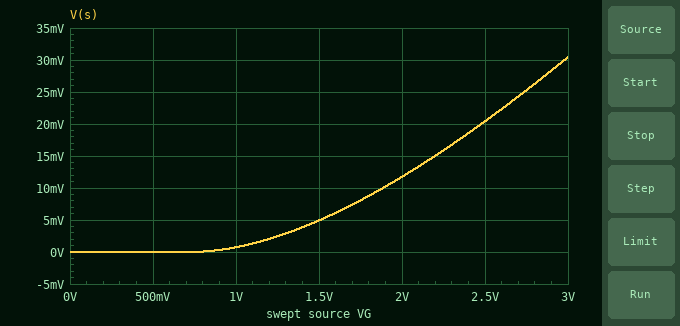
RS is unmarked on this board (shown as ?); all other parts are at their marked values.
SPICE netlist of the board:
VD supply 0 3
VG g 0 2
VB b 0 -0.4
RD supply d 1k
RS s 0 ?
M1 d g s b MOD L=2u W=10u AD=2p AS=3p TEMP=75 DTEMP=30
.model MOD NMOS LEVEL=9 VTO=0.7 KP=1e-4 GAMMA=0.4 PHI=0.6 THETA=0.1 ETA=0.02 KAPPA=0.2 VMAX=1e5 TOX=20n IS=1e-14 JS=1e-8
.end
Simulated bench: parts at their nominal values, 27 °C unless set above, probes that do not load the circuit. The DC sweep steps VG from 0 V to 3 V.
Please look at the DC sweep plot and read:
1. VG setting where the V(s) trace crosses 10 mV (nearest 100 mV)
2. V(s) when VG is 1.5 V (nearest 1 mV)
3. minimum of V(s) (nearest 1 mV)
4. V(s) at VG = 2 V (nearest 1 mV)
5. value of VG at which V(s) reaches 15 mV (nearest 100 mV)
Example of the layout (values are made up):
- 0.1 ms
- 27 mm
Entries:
- 1.9 V
- 5 mV
- 0 V
- 12 mV
- 2.2 V
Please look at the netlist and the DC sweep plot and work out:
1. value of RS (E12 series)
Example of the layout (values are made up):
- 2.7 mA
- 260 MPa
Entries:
- 56 Ω
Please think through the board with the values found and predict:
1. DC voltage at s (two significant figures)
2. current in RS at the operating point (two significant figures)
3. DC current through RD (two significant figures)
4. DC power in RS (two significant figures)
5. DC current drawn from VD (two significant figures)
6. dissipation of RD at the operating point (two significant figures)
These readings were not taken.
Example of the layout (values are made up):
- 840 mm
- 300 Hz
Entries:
- 12 mV
- 210 µA
- 210 µA
- 2.5 µW
- 210 µA
- 44 µW
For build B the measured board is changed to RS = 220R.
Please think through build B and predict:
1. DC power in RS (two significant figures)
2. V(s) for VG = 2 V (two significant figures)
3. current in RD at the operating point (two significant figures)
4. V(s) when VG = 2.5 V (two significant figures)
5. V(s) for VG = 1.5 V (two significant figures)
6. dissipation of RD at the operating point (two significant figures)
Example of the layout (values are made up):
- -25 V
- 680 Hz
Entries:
- 8.7 µW
- 44 mV
- 200 µA
- 75 mV
- 19 mV
- 40 µW
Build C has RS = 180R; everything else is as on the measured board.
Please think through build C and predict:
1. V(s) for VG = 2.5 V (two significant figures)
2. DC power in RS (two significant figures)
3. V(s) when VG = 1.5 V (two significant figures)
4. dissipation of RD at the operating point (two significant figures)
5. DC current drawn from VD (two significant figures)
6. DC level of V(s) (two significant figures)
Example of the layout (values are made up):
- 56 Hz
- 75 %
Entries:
- 63 mV
- 7.3 µW
- 15 mV
- 41 µW
- 200 µA
- 36 mV
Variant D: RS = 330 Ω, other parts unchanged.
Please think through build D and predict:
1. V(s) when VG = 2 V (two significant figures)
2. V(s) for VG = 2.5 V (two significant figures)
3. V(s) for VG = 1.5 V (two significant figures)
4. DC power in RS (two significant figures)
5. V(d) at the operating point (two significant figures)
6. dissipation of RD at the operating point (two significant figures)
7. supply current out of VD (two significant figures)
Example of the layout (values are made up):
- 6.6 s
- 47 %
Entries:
- 64 mV
- 110 mV
- 27 mV
- 12 µW
- 2.8 V
- 37 µW
- 190 µA
